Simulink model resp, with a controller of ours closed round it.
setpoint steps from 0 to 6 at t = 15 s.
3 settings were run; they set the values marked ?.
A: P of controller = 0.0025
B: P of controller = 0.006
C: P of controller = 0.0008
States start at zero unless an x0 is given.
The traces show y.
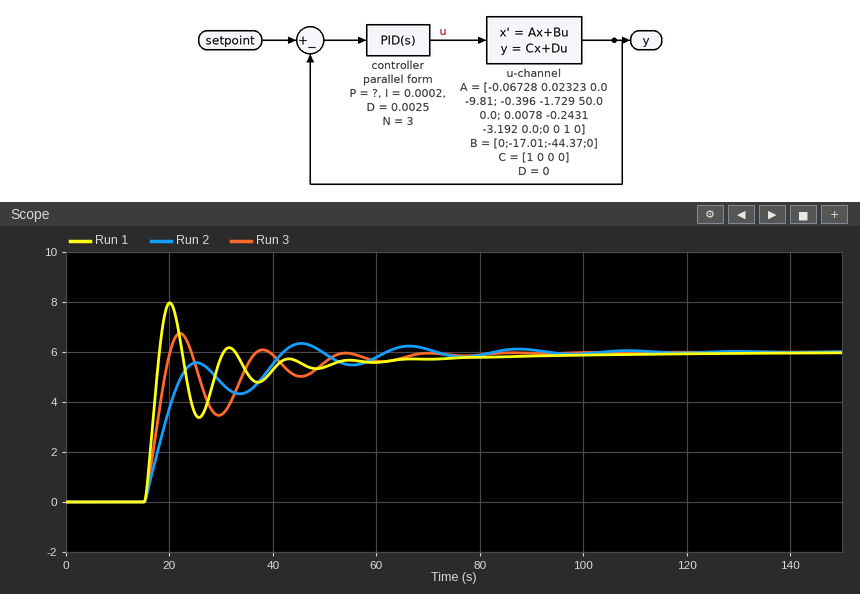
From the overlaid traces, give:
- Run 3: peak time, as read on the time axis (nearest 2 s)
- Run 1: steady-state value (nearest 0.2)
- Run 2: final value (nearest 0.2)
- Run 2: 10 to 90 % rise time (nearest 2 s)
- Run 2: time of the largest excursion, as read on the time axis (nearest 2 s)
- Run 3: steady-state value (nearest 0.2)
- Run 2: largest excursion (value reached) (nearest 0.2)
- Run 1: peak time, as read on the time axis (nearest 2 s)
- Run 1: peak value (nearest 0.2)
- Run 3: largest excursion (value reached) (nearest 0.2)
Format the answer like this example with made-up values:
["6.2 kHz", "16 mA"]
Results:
["22 s", "6.0", "6.0", "8 s", "46 s", "6.0", "6.4", "20 s", "8.0", "6.8"]
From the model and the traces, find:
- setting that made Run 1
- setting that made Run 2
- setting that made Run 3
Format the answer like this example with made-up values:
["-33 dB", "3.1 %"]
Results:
["B", "C", "A"]
